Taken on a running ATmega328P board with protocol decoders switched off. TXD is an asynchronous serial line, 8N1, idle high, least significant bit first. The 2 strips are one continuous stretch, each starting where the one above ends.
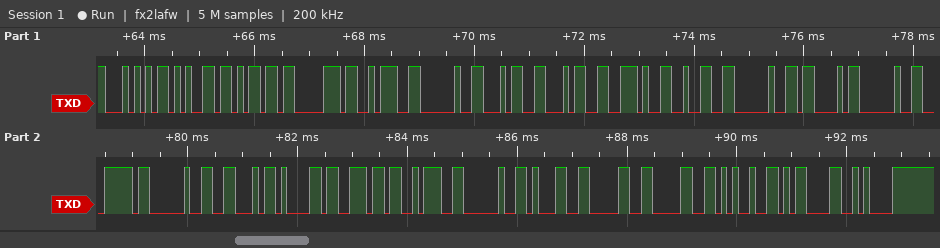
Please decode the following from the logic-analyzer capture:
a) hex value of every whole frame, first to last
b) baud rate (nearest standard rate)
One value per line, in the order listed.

0x54 0x65 0x6D 0x70 0x3A 0x20 0x34 0x34 0x2E 0x32 0x20 0x43 0x20 0x7C 0x20 0x46 0x61 0x6E 0x3A 0x20 0x31 0x30 0x30 0x25 0x0D 0x0A
9600 baud
